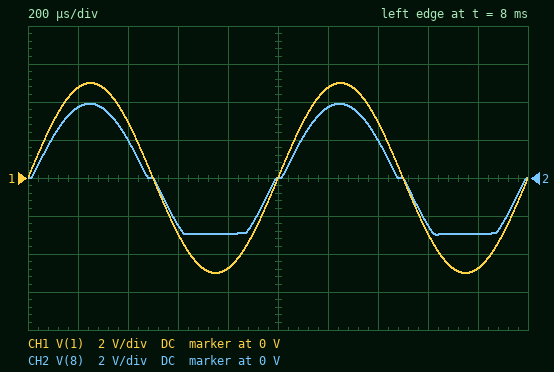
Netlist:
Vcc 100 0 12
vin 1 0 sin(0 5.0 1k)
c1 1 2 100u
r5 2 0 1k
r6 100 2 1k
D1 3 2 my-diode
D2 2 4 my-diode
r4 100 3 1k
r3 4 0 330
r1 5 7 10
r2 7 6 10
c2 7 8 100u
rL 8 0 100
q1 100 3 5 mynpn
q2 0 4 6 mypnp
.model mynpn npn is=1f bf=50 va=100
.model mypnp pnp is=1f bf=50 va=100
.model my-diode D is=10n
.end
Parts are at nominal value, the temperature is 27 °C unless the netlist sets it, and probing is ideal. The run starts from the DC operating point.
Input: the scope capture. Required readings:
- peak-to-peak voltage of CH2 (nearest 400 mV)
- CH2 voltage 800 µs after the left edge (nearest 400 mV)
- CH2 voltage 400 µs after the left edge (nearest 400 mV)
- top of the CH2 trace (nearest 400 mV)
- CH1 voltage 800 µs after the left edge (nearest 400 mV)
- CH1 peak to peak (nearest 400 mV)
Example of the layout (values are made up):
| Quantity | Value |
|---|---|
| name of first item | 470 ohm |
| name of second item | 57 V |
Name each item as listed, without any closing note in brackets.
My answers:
| Quantity | Value |
|---|---|
| peak-to-peak voltage of CH2 | 6.8 V |
| CH2 voltage 800 µs after the left edge | -2.8 V |
| CH2 voltage 400 µs after the left edge | 2.0 V |
| top of the CH2 trace | 4.0 V |
| CH1 voltage 800 µs after the left edge | -4.8 V |
| CH1 peak to peak | 10.0 V |
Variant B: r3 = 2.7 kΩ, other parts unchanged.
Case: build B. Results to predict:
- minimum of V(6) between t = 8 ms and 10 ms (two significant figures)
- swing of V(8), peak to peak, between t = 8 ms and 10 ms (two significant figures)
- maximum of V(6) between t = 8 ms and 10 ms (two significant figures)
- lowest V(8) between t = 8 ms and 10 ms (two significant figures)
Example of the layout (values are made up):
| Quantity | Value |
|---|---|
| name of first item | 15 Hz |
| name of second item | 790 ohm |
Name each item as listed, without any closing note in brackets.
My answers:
| Quantity | Value |
|---|---|
| minimum of V(6) between t = 8 ms and 10 ms | 2.8 V |
| swing of V(8), peak to peak, between t = 8 ms and 10 ms | 7.1 V |
| maximum of V(6) between t = 8 ms and 10 ms | 10 V |
| lowest V(8) between t = 8 ms and 10 ms | -3.8 V |
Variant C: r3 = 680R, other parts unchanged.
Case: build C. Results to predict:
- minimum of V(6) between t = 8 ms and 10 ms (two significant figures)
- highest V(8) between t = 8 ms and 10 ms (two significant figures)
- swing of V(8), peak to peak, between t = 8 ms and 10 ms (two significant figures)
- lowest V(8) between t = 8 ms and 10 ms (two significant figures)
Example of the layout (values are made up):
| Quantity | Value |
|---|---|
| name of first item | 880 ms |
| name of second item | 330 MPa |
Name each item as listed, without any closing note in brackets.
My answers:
| Quantity | Value |
|---|---|
| minimum of V(6) between t = 8 ms and 10 ms | 1.3 V |
| highest V(8) between t = 8 ms and 10 ms | 4.0 V |
| swing of V(8), peak to peak, between t = 8 ms and 10 ms | 7.8 V |
| lowest V(8) between t = 8 ms and 10 ms | -3.8 V |
